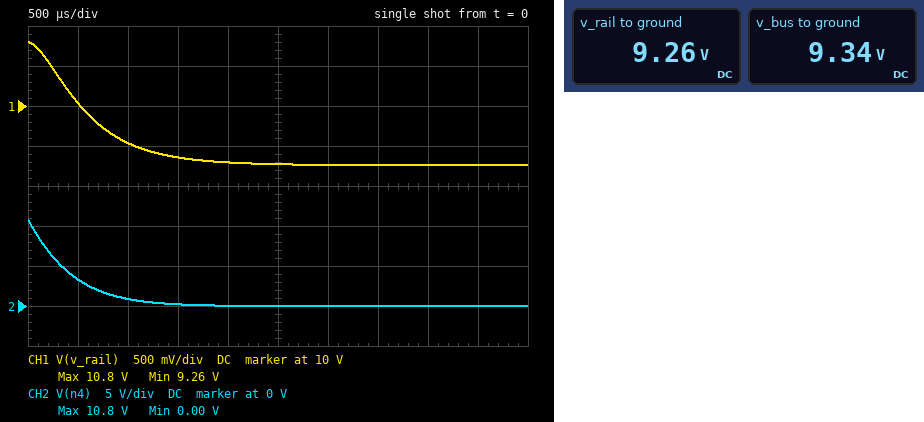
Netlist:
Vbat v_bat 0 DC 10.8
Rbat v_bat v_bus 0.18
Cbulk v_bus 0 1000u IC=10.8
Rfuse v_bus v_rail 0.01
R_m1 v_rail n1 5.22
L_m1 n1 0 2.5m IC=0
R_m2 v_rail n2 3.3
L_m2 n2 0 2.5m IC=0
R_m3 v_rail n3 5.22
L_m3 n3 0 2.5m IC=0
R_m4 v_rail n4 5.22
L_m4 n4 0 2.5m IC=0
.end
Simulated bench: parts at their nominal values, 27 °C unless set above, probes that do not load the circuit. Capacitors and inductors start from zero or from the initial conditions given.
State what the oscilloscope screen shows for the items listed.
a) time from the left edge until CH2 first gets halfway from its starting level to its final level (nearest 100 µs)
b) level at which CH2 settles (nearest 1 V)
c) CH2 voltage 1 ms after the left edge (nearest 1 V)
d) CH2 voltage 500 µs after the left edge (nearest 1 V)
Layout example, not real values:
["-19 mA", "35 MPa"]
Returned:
["300 µs", "0 V", "1 V", "3 V"]
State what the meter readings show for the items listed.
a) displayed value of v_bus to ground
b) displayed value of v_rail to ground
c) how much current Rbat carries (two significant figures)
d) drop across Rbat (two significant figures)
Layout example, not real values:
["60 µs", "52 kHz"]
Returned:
["9.34 V", "9.26 V", "8.1 A", "1.5 V"]
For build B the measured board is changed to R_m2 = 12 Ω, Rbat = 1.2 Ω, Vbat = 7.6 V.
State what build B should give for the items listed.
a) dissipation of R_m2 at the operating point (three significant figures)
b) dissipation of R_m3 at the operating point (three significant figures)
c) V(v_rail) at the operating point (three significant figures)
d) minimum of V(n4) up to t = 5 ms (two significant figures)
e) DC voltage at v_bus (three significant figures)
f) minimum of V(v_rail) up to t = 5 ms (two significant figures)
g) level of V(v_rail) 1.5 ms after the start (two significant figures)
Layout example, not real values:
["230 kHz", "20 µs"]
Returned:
["1.49 W", "3.43 W", "4.23 V", "-930 mV", "4.26 V", "4.2 V", "5.0 V"]
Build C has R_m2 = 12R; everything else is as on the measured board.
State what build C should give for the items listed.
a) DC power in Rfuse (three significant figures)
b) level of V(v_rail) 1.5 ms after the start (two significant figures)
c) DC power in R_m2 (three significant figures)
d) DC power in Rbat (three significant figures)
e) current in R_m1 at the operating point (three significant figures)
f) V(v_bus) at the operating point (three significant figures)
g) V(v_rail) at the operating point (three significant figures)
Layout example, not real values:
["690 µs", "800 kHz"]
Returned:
["399 mW", "9.6 V", "7.68 W", "7.18 W", "1.84 A", "9.66 V", "9.60 V"]
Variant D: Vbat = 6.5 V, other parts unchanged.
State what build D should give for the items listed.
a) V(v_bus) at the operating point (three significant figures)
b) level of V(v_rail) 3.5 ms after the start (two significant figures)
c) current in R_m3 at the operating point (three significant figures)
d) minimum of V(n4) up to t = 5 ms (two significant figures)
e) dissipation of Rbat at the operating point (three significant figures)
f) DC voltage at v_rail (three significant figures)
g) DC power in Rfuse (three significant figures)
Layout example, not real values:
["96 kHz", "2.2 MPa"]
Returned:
["5.62 V", "5.6 V", "1.07 A", "-4.6 mV", "4.30 W", "5.57 V", "239 mW"]
